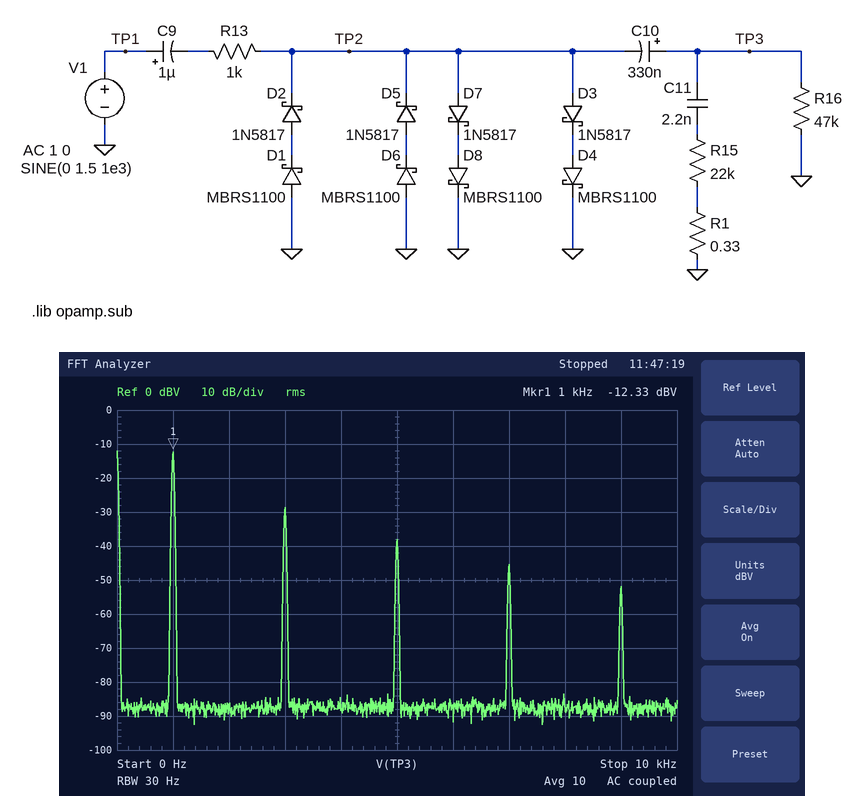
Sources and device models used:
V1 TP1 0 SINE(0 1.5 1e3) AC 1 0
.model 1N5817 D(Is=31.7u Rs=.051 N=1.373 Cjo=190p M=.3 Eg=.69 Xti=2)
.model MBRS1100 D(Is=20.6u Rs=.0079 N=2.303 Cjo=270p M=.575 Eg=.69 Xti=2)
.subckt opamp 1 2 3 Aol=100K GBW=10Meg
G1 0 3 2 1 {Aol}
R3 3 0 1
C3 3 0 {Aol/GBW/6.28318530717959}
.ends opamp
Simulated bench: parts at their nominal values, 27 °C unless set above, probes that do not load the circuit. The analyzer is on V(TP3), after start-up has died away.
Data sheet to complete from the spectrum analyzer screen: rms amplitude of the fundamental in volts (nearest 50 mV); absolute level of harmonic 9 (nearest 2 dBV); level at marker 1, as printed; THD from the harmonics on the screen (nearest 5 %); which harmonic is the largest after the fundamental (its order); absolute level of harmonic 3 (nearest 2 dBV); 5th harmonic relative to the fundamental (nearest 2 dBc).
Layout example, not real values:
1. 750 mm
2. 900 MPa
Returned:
1. 250 mV
2. -52 dBV
3. -12.33 dBV
4. 15 %
5. 3
6. -28 dBV
7. -26 dBc
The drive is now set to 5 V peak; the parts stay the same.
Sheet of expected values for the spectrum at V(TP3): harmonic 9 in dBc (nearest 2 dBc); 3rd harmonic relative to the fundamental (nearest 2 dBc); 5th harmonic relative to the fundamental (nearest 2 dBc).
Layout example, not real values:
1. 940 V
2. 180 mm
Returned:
1. -28 dBc
2. -14 dBc
3. -20 dBc
